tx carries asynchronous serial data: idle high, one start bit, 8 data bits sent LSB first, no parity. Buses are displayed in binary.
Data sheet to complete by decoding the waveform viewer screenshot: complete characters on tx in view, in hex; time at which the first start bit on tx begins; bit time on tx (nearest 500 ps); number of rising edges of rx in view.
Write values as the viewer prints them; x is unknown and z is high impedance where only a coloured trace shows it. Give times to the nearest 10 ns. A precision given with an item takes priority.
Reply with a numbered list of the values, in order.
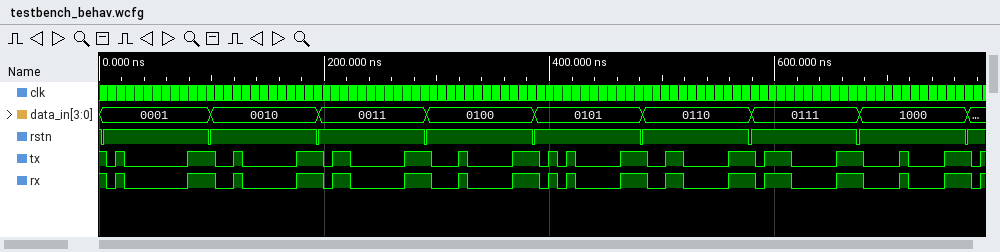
1. 01, 02, 03, 04, 05, 06, 07, 08
2. 10 ns
3. 8000 ps
4. 18
